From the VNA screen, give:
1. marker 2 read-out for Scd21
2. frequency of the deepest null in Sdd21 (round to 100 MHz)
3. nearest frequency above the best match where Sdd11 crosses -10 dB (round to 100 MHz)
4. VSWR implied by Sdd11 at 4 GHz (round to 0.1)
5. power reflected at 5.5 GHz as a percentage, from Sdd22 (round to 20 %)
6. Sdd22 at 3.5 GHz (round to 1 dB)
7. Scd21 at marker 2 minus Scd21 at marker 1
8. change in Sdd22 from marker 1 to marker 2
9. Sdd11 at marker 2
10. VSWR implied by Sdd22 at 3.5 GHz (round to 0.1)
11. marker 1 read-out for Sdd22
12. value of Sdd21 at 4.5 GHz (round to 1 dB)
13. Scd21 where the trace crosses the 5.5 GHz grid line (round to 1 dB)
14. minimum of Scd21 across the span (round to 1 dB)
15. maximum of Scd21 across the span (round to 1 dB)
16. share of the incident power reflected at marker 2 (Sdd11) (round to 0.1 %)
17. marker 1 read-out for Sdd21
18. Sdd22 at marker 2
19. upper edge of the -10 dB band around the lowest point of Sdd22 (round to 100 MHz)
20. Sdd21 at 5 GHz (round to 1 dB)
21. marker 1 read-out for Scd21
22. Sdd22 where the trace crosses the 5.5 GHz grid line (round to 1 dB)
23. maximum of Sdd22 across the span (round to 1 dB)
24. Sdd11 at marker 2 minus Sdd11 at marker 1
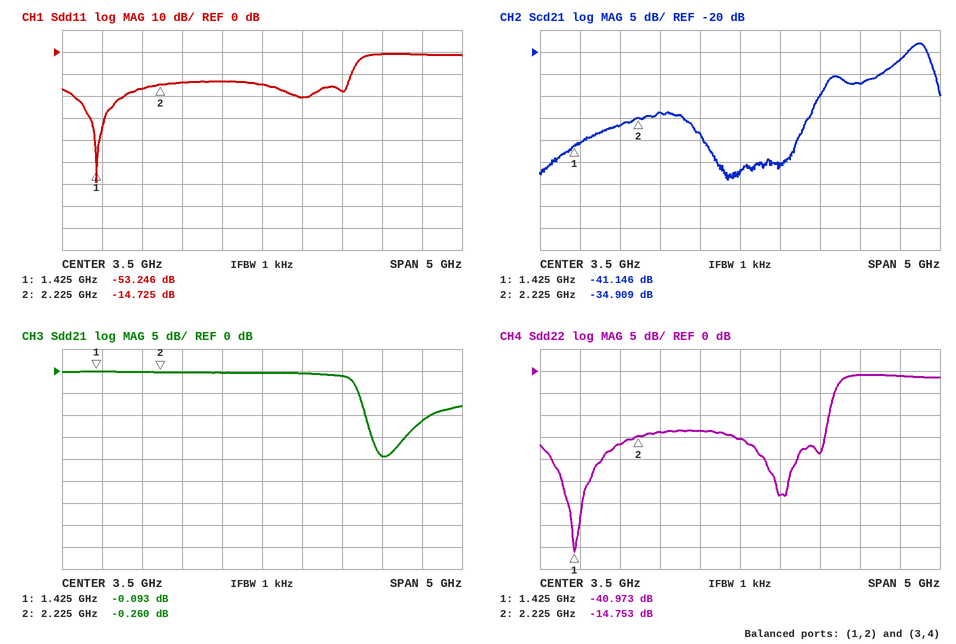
-34.909 dB
5.0 GHz
4.6 GHz
1.2
80 %
-15 dB
6.237 dB
26.220 dB
-14.725 dB
1.4
-40.973 dB
-1 dB
-22 dB
-49 dB
-18 dB
3.4 %
-0.093 dB
-14.753 dB
4.6 GHz
-19 dB
-41.146 dB
-1 dB
-1 dB
38.521 dB
